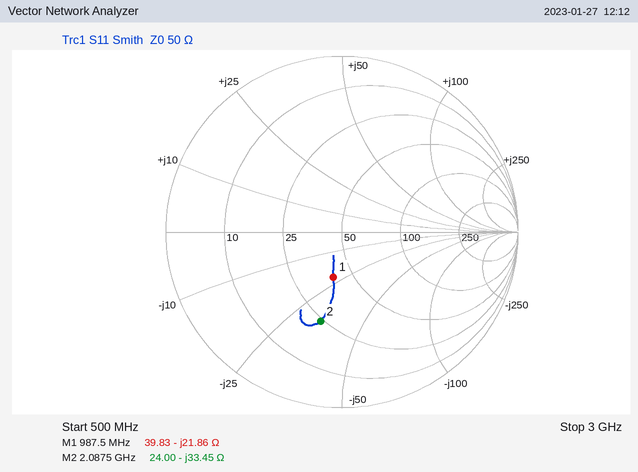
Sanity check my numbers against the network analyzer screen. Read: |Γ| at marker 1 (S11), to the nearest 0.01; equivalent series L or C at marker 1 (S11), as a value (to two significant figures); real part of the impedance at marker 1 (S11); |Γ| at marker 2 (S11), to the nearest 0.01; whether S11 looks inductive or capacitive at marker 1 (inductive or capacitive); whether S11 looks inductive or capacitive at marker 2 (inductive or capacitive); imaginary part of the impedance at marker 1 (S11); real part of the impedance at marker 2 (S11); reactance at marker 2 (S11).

0.26
7.4 pF
39.83 Ω
0.52
capacitive
capacitive
-21.86 Ω
24.00 Ω
-33.45 Ω
